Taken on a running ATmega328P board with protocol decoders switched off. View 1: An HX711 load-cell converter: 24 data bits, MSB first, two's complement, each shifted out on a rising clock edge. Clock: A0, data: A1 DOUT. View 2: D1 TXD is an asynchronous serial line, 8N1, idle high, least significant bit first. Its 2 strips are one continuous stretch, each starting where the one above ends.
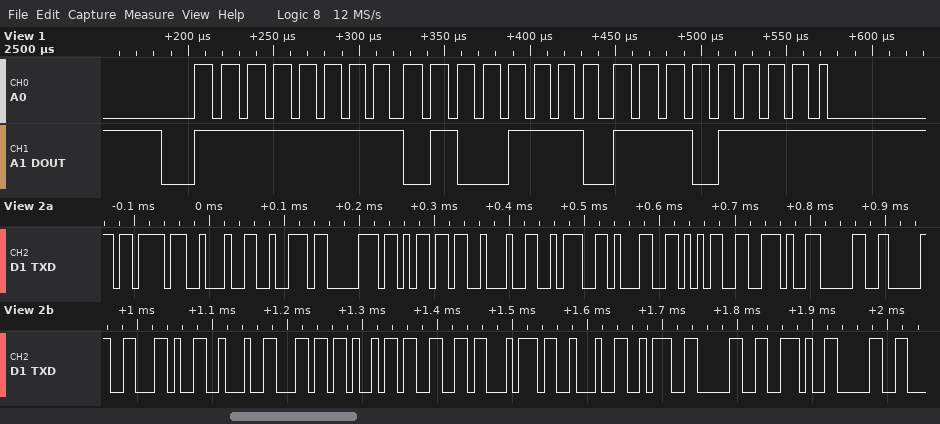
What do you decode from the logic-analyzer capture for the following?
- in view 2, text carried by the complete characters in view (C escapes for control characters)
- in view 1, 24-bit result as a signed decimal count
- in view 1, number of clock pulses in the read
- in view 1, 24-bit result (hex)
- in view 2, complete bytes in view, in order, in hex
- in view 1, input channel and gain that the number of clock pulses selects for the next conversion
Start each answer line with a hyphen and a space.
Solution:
- "{\"rpm\":15.00,\"lift\":0.0"
- -45329
- 25
- 0xFF4EEF
- 7B 22 72 70 6D 22 3A 31 35 2E 30 30 2C 22 6C 69 66 74 22 3A 30 2E 30
- channel A, gain 128
